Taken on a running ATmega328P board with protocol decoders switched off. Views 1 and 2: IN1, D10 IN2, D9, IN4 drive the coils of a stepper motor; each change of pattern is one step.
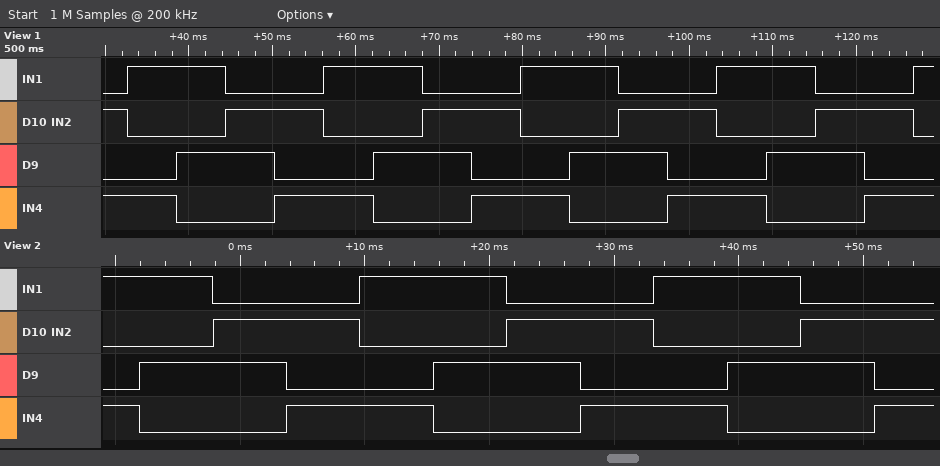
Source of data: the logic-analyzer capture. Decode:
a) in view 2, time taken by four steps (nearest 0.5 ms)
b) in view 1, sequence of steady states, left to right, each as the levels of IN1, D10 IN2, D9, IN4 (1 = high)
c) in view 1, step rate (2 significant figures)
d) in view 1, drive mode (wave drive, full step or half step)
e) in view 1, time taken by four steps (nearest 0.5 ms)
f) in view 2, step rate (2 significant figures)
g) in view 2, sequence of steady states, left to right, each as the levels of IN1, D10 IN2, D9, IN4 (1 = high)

23.5 ms
0101 1001 1010 0110 0101 1001 1010 0110 0101 1001 1010 0110 0101 1001 1010 0110 0101 1001
170 steps/s
full step
23.5 ms
170 steps/s
1001 1010 0110 0101 1001 1010 0110 0101 1001 1010 0110 0101
